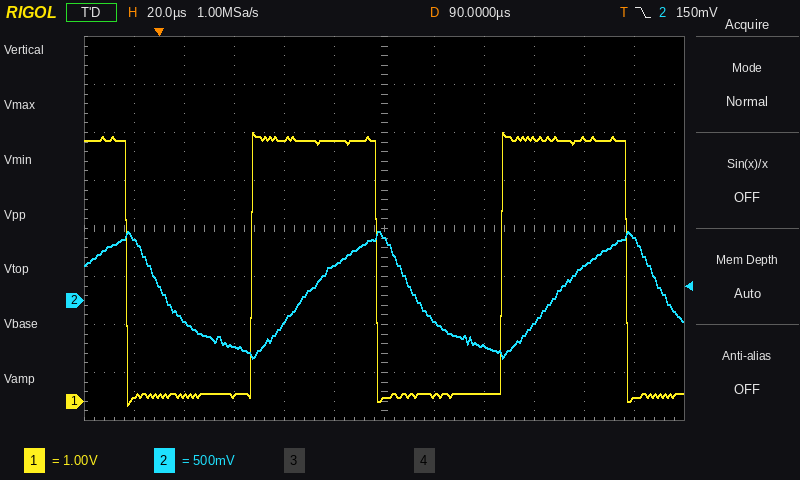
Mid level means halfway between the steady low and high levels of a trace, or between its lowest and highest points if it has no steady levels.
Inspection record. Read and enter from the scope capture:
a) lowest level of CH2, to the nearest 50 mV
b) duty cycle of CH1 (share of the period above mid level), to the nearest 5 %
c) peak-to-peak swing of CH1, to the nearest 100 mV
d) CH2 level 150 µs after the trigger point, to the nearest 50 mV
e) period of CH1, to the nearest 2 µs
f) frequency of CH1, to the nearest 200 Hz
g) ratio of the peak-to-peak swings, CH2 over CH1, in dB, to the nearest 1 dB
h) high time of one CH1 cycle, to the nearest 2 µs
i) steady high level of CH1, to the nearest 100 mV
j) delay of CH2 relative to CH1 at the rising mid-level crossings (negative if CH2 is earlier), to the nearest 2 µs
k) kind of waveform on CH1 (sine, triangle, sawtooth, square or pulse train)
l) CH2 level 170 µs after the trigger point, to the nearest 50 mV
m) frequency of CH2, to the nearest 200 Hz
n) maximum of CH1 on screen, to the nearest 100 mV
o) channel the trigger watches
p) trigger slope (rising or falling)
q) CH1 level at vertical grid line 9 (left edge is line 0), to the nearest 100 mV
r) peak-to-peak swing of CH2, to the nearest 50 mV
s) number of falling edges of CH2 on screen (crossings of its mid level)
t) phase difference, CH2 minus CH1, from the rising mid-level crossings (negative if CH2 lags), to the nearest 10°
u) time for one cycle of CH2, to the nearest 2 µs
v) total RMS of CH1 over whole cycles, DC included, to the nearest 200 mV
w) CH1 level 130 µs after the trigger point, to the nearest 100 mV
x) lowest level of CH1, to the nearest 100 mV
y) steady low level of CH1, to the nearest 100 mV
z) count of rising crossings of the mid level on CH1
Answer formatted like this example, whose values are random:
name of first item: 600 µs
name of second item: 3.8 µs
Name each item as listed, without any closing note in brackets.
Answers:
lowest level of CH2, to the nearest 50 mV: -600 mV
duty cycle of CH1 (share of the period above mid level), to the nearest 5 %: 50 %
peak-to-peak swing of CH1, to the nearest 100 mV: 5.7 V
CH2 level 150 µs after the trigger point, to the nearest 50 mV: -250 mV
period of CH1, to the nearest 2 µs: 100 µs
frequency of CH1, to the nearest 200 Hz: 10.0 kHz
ratio of the peak-to-peak swings, CH2 over CH1, in dB, to the nearest 1 dB: -13 dB
high time of one CH1 cycle, to the nearest 2 µs: 50 µs
steady high level of CH1, to the nearest 100 mV: 5.4 V
delay of CH2 relative to CH1 at the rising mid-level crossings (negative if CH2 is earlier), to the nearest 2 µs: +22 µs
kind of waveform on CH1: square
CH2 level 170 µs after the trigger point, to the nearest 50 mV: 350 mV
frequency of CH2, to the nearest 200 Hz: 10.0 kHz
maximum of CH1 on screen, to the nearest 100 mV: 5.6 V
channel the trigger watches: CH2
trigger slope: falling
CH1 level at vertical grid line 9 (left edge is line 0), to the nearest 100 mV: 5.5 V
peak-to-peak swing of CH2, to the nearest 50 mV: 1.30 V
number of falling edges of CH2 on screen: 3
phase difference, CH2 minus CH1, from the rising mid-level crossings (negative if CH2 lags), to the nearest 10°: -80°
time for one cycle of CH2, to the nearest 2 µs: 100 µs
total RMS of CH1 over whole cycles, DC included, to the nearest 200 mV: 3.8 V
CH1 level 130 µs after the trigger point, to the nearest 100 mV: 200 mV
lowest level of CH1, to the nearest 100 mV: -100 mV
steady low level of CH1, to the nearest 100 mV: 200 mV
count of rising crossings of the mid level on CH1: 2
